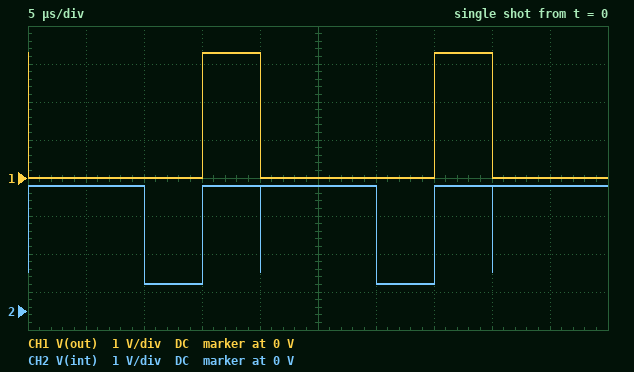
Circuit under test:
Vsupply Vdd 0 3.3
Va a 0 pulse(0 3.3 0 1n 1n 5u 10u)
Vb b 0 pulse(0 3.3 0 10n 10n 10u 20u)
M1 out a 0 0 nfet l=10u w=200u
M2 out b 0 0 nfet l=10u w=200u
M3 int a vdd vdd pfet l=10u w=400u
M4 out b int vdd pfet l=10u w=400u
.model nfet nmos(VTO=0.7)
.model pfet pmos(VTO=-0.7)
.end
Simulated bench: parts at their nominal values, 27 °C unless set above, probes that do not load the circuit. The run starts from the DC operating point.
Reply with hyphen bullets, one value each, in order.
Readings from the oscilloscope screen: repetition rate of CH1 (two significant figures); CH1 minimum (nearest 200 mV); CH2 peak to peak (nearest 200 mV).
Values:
- 50 kHz
- 0 V
- 2.6 V
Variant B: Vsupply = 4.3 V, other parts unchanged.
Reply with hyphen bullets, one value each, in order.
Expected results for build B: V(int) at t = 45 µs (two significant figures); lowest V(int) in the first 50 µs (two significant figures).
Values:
- 4.2 V
- 1.0 V
